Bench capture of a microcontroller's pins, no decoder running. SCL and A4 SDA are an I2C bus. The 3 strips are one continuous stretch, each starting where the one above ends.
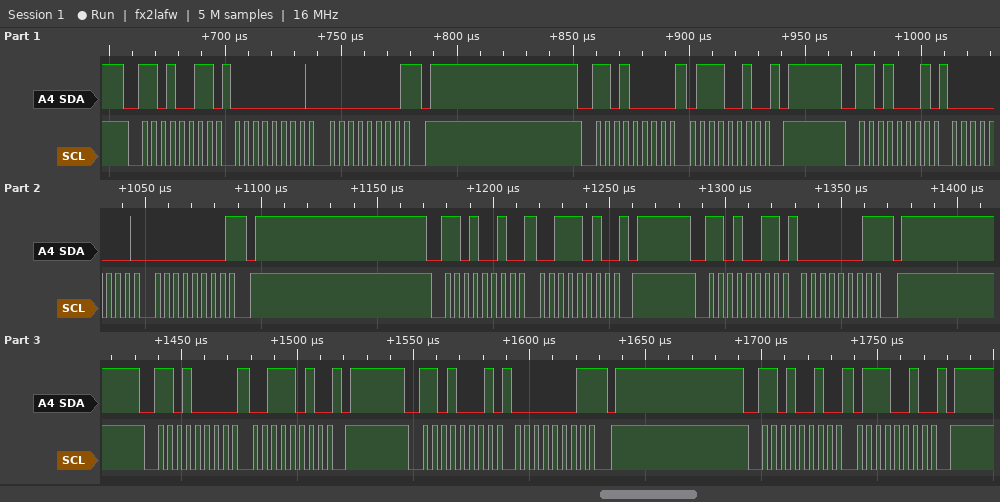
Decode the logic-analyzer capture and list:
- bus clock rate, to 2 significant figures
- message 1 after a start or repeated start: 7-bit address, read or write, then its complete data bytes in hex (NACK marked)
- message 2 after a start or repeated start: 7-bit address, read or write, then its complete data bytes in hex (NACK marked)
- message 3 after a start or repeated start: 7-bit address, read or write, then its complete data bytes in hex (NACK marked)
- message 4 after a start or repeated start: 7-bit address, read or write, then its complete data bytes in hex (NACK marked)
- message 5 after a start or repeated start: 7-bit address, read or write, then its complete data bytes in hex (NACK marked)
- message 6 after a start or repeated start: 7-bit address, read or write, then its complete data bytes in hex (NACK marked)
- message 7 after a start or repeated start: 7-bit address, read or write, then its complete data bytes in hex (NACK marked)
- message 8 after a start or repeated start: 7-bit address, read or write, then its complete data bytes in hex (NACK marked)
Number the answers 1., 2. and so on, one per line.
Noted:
1. 250 kHz
2. 0x69 read: 00 00 NACK
3. 0x68 write: 72
4. 0x68 read: 00 00 NACK
5. 0x69 write: 3A
6. 0x69 read: 01 NACK
7. 0x68 write: 3A
8. 0x68 read: 01 NACK
9. 0x69 write: 72
